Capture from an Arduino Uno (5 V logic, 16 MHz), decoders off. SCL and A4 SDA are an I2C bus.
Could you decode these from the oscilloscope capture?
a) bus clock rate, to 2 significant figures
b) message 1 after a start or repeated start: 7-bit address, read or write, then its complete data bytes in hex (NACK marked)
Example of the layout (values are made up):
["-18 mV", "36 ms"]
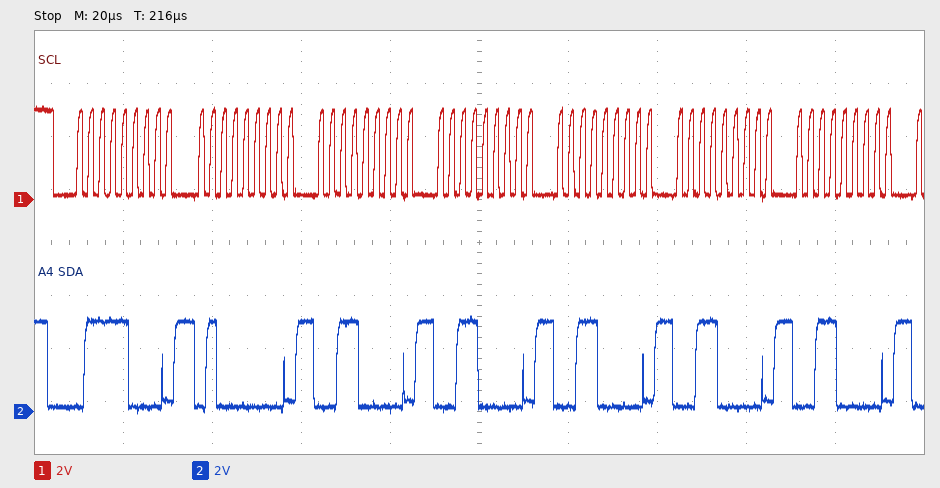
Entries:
["400 kHz", "0x3C write: 40 30 30 30 30 30"]
